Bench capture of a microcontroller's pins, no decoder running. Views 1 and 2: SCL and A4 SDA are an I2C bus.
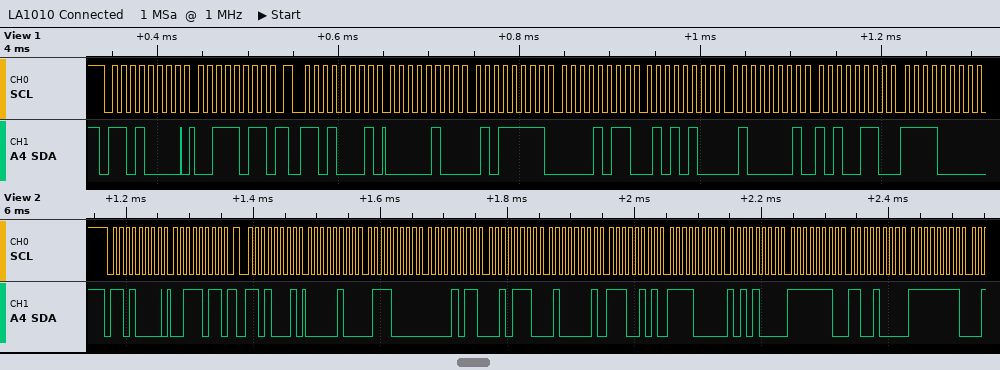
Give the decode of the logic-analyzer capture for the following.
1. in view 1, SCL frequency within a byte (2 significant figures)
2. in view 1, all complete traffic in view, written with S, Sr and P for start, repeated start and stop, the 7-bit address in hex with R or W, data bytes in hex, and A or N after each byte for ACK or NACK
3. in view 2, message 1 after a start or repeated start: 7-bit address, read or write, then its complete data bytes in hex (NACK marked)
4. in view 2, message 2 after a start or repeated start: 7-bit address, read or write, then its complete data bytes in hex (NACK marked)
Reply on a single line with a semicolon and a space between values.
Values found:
100 kHz; S 68W A 3B A Sr 68R A 04 A 5F A 0B A 54 A 41 A A6 A F0 A; 0x68 write: 3B; 0x68 read: 04 70 0B 2E 41 E5 F0 A8 FE C8 FF
